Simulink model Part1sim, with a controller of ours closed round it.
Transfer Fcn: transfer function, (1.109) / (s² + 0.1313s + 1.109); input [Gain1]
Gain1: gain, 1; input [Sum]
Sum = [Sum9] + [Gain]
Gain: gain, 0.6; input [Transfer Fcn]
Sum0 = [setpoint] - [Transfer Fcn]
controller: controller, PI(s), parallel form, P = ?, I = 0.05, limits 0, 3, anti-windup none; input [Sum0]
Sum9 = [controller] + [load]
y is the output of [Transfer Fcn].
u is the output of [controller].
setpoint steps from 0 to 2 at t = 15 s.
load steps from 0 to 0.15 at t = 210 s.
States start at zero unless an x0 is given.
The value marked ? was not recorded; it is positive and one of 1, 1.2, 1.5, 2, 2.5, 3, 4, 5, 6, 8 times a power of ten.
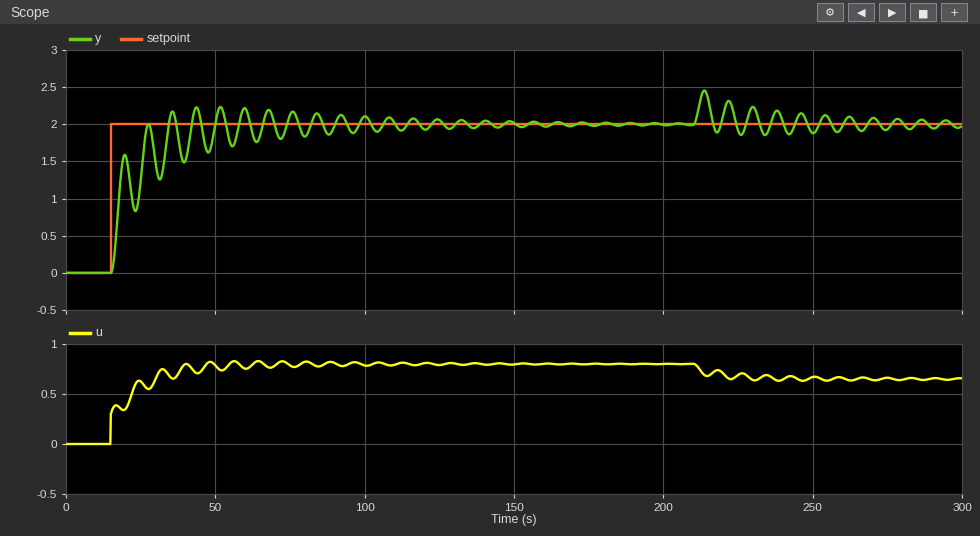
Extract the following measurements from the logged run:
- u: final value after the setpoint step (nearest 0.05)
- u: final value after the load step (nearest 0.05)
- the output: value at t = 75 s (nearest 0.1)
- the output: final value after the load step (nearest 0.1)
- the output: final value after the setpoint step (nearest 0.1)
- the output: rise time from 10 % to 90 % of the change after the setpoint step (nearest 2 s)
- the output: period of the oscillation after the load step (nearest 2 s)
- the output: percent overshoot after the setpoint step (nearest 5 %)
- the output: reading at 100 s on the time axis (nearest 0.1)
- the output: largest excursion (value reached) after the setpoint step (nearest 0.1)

0.80
0.65
2.1
2.0
2.0
10 s
8 s
10 %
2.1
2.2
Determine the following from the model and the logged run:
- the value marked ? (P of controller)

0.15
